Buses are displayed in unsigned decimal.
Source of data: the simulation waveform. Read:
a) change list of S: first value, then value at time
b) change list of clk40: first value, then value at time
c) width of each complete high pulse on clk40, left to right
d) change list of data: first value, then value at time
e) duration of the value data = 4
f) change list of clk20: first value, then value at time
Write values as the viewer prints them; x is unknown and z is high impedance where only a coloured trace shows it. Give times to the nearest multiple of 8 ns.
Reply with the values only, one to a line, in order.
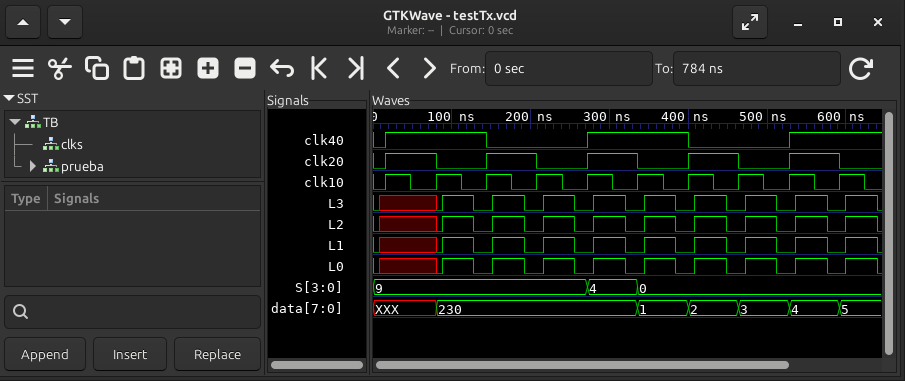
9, 4 at 272 ns, 0 at 336 ns
0, 1 at 16 ns, 0 at 144 ns, 1 at 272 ns, 0 at 400 ns, 1 at 528 ns
128 ns, 128 ns
XXX, 230 at 80 ns, 1 at 336 ns, 2 at 400 ns, 3 at 464 ns, 4 at 528 ns, 5 at 592 ns
64 ns
0, 1 at 16 ns, 0 at 80 ns, 1 at 144 ns, 0 at 208 ns, 1 at 272 ns, 0 at 336 ns, 1 at 400 ns, 0 at 464 ns, 1 at 528 ns, 0 at 592 ns
